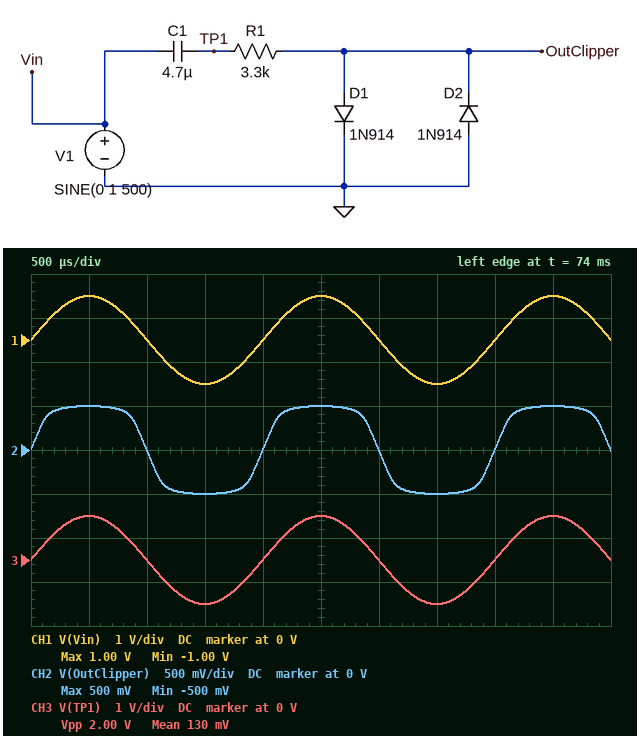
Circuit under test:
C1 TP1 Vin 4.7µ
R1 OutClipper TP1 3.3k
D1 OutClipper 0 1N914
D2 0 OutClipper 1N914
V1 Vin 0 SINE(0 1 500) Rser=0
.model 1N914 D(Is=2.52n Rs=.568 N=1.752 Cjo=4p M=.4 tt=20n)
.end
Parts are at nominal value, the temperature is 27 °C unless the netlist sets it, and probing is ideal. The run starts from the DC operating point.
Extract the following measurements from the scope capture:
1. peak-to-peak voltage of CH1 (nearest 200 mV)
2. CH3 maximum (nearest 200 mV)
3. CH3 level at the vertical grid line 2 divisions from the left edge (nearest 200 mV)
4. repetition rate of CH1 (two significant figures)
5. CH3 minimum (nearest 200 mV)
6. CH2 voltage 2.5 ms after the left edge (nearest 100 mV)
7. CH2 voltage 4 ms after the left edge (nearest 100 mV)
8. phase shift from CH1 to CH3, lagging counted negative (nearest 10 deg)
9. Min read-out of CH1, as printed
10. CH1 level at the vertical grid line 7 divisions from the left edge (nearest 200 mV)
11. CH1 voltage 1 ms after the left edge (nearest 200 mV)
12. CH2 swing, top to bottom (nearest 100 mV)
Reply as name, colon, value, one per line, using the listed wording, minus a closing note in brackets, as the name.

peak-to-peak voltage of CH1: 2.0 V
CH3 maximum: 1.0 V
CH3 level at the vertical grid line 2 divisions from the left edge: 0 V
repetition rate of CH1: 500 Hz
CH3 minimum: -1.0 V
CH2 voltage 2.5 ms after the left edge: 500 mV
CH2 voltage 4 ms after the left edge: 0 V
phase shift from CH1 to CH3, lagging counted negative: 0 deg
Min read-out of CH1, as printed: -1.00 V
CH1 level at the vertical grid line 7 divisions from the left edge: -1.0 V
CH1 voltage 1 ms after the left edge: 0 V
CH2 swing, top to bottom: 1.0 V
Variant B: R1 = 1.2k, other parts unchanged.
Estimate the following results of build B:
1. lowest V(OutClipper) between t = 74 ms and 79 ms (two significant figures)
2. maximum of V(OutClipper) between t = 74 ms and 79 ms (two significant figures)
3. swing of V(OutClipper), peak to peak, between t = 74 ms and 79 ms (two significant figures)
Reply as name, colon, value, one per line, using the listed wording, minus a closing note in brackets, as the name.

lowest V(OutClipper) between t = 74 ms and 79 ms: -540 mV
maximum of V(OutClipper) between t = 74 ms and 79 ms: 540 mV
swing of V(OutClipper), peak to peak, between t = 74 ms and 79 ms: 1.1 V
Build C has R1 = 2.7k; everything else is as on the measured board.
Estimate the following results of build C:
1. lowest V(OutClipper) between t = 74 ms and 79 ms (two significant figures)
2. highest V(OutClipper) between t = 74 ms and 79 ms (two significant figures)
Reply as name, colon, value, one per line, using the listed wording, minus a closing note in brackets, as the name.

lowest V(OutClipper) between t = 74 ms and 79 ms: -510 mV
highest V(OutClipper) between t = 74 ms and 79 ms: 510 mV
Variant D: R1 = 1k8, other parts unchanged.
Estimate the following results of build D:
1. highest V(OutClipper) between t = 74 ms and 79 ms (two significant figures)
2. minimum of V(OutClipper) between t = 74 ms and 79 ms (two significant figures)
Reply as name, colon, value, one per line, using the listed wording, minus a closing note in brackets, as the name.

highest V(OutClipper) between t = 74 ms and 79 ms: 520 mV
minimum of V(OutClipper) between t = 74 ms and 79 ms: -520 mV
